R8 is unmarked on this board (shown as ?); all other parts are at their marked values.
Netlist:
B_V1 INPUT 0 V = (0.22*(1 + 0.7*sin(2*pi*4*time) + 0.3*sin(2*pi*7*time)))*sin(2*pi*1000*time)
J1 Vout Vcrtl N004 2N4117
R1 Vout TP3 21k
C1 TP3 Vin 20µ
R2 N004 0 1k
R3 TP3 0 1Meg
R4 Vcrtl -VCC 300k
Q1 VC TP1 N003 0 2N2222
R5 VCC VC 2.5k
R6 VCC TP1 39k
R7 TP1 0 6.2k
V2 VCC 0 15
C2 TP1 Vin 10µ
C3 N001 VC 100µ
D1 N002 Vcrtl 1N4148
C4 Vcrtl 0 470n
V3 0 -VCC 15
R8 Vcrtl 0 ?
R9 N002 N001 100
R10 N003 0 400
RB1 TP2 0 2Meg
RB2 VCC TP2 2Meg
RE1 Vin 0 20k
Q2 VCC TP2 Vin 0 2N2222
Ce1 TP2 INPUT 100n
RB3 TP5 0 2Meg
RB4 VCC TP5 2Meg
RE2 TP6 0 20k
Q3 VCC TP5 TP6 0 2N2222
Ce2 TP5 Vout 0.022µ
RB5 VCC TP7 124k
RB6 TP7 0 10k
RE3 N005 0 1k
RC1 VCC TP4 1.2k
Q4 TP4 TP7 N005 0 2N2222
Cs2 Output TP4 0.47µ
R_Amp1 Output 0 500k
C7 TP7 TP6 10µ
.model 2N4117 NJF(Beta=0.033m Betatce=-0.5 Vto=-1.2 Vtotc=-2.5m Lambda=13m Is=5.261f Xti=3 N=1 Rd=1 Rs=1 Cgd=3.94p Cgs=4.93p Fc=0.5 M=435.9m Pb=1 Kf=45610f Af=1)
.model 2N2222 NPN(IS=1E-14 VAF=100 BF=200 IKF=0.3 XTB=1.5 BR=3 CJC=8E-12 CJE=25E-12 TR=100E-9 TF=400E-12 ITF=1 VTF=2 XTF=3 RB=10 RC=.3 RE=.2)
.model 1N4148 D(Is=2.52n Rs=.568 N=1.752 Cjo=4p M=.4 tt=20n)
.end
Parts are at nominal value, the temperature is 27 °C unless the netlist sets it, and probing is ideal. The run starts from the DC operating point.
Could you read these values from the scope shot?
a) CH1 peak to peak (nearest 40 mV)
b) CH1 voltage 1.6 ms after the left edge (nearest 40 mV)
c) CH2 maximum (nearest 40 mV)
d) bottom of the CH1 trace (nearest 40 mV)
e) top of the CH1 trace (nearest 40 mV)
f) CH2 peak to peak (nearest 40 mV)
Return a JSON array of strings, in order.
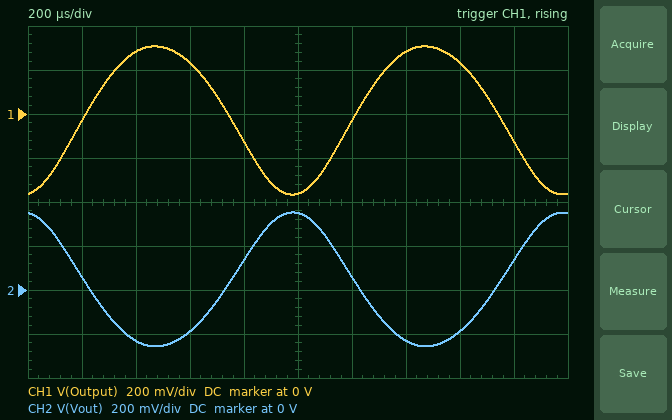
["680 mV", "240 mV", "360 mV", "-360 mV", "320 mV", "600 mV"]
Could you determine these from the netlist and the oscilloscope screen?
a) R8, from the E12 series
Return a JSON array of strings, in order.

["56 kΩ"]
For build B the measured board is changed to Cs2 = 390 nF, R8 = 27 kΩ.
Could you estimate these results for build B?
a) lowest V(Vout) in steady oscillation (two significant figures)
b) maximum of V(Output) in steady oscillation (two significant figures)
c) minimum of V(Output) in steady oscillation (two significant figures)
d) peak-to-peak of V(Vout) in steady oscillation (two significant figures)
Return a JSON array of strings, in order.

["-150 mV", "170 mV", "-180 mV", "320 mV"]
